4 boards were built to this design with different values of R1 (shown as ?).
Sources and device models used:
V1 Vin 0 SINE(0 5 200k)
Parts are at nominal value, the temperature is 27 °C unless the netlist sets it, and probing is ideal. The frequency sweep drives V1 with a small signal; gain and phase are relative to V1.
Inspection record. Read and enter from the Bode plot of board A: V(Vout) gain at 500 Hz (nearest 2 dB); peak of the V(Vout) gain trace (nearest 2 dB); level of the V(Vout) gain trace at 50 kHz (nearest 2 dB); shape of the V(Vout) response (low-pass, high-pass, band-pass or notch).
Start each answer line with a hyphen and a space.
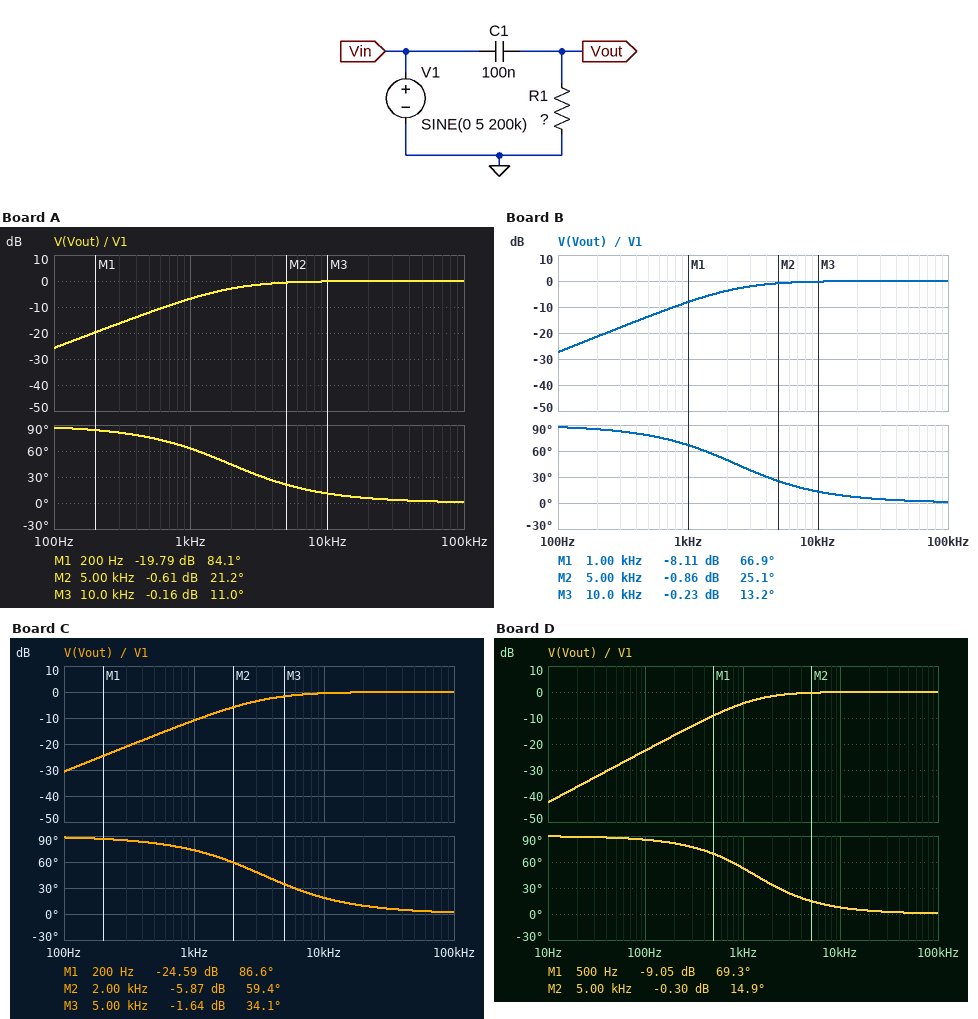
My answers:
- -12 dB
- 0 dB
- 0 dB
- high-pass
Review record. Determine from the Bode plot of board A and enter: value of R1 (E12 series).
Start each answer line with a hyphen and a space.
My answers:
- 820 Ω
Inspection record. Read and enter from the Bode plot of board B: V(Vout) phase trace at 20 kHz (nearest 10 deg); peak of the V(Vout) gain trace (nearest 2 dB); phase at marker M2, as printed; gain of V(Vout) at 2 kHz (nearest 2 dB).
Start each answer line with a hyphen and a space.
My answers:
- 10 deg
- 0 dB
- 25.1 deg
- -4 dB
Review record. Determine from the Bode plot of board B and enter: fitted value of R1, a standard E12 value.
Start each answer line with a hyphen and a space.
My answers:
- 680 Ω
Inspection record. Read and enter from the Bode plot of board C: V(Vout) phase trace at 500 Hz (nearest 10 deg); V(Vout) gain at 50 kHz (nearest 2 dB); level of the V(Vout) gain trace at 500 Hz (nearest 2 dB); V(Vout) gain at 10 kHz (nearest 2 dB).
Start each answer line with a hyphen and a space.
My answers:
- 80 deg
- 0 dB
- -16 dB
- 0 dB
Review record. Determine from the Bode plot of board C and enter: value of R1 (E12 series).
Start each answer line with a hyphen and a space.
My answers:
- 470 Ω
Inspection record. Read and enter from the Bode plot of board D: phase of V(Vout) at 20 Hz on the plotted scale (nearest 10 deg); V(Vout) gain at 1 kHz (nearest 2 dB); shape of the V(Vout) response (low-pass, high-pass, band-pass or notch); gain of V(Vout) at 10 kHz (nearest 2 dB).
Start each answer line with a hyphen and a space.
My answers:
- 90 deg
- -4 dB
- high-pass
- 0 dB
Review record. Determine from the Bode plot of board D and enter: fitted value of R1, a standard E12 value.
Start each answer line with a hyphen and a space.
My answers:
- 1.2 kΩ
